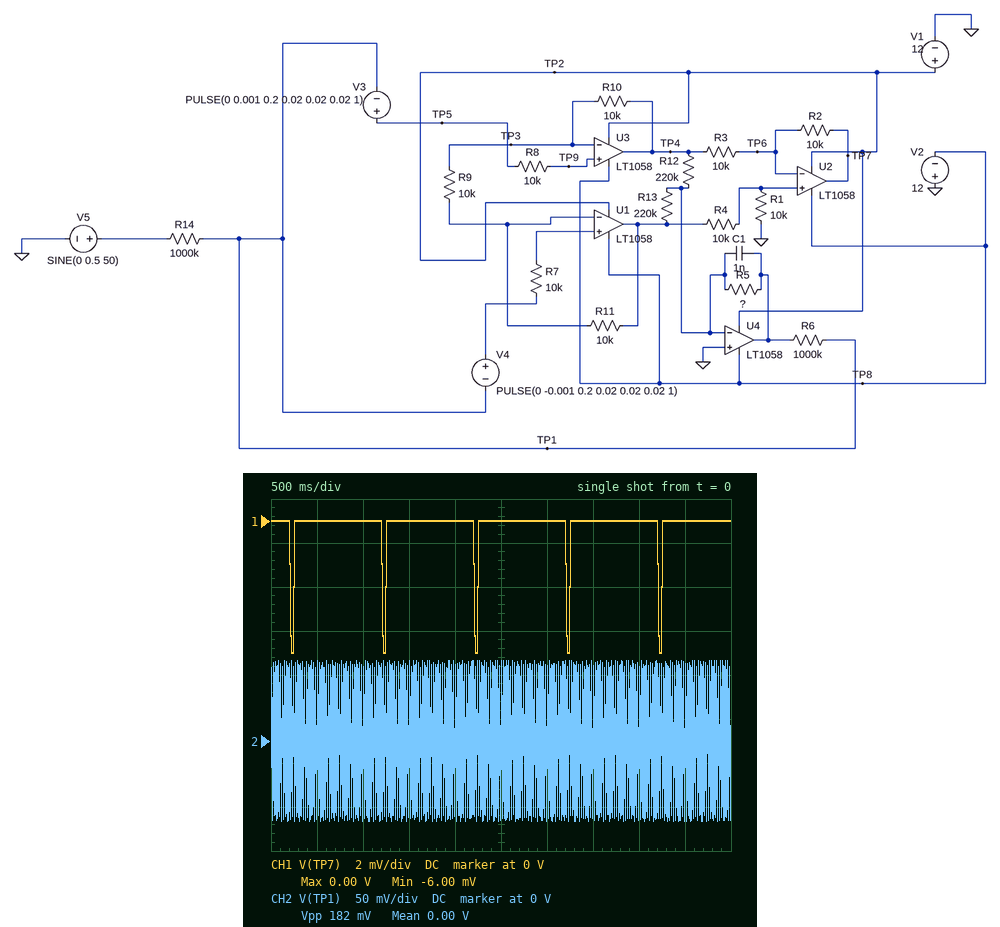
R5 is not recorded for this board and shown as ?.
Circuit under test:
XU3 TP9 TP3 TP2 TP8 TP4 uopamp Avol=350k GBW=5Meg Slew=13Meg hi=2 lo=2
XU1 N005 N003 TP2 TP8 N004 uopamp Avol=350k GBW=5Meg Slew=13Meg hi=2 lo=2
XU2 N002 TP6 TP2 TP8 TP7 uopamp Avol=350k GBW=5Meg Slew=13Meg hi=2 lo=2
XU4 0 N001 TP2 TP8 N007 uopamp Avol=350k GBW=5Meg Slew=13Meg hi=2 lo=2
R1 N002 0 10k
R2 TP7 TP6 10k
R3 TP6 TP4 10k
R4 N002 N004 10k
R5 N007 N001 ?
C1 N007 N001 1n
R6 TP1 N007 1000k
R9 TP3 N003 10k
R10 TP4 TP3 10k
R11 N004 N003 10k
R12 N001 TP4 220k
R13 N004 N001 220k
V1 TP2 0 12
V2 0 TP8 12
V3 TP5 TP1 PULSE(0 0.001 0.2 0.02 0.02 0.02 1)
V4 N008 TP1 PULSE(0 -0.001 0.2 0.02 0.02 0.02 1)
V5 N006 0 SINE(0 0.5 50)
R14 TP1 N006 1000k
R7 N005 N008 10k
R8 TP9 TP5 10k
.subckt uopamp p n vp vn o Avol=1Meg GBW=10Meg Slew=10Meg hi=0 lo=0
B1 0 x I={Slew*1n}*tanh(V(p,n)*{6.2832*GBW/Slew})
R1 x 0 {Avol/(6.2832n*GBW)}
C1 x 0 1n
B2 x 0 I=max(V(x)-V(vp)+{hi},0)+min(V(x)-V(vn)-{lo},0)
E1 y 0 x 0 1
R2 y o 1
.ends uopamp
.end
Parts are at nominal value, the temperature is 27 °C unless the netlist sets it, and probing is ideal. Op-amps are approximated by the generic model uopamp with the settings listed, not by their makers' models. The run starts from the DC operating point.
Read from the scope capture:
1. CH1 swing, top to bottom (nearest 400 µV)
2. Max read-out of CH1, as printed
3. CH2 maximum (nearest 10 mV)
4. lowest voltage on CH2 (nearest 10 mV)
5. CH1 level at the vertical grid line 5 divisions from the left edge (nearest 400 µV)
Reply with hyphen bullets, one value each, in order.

- 6.0 mV
- 0.00 V
- 90 mV
- -90 mV
- 0 V
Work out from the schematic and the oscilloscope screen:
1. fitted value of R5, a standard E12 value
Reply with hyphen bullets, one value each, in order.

- 390 kΩ
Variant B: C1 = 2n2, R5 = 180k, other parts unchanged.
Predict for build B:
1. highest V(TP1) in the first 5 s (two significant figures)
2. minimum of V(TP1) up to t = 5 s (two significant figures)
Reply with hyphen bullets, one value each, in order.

- 140 mV
- -140 mV
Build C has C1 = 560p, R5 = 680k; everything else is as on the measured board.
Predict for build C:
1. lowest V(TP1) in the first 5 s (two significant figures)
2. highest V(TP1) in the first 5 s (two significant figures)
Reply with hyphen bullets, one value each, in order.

- -62 mV
- 62 mV
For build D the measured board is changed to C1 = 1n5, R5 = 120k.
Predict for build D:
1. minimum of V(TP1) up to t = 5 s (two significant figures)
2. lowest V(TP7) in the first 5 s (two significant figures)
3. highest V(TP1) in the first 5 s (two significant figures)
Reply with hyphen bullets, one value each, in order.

- -160 mV
- -6.0 mV
- 160 mV
